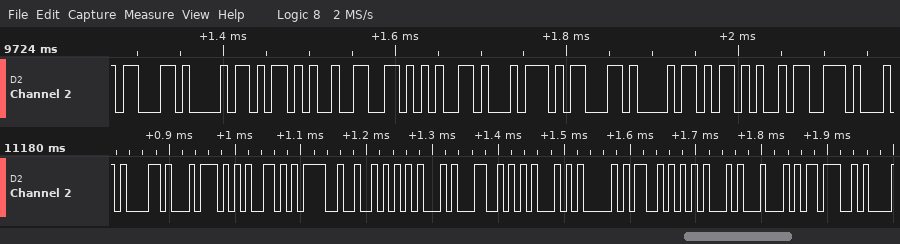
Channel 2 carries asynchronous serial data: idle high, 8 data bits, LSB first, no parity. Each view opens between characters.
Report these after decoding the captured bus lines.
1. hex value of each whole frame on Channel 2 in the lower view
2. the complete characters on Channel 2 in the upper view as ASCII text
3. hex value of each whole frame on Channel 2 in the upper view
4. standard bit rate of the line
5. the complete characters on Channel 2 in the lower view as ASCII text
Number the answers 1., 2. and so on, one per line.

1. 61, 74, 65, 3D, 52, 45, 4C, 45, 41, 53, 45, 44, 3B
2. "ch+fetch+s"
3. 63, 68, 2B, 66, 65, 74, 63, 68, 2B, 73
4. 115200 baud
5. "ate=RELEASED;"
